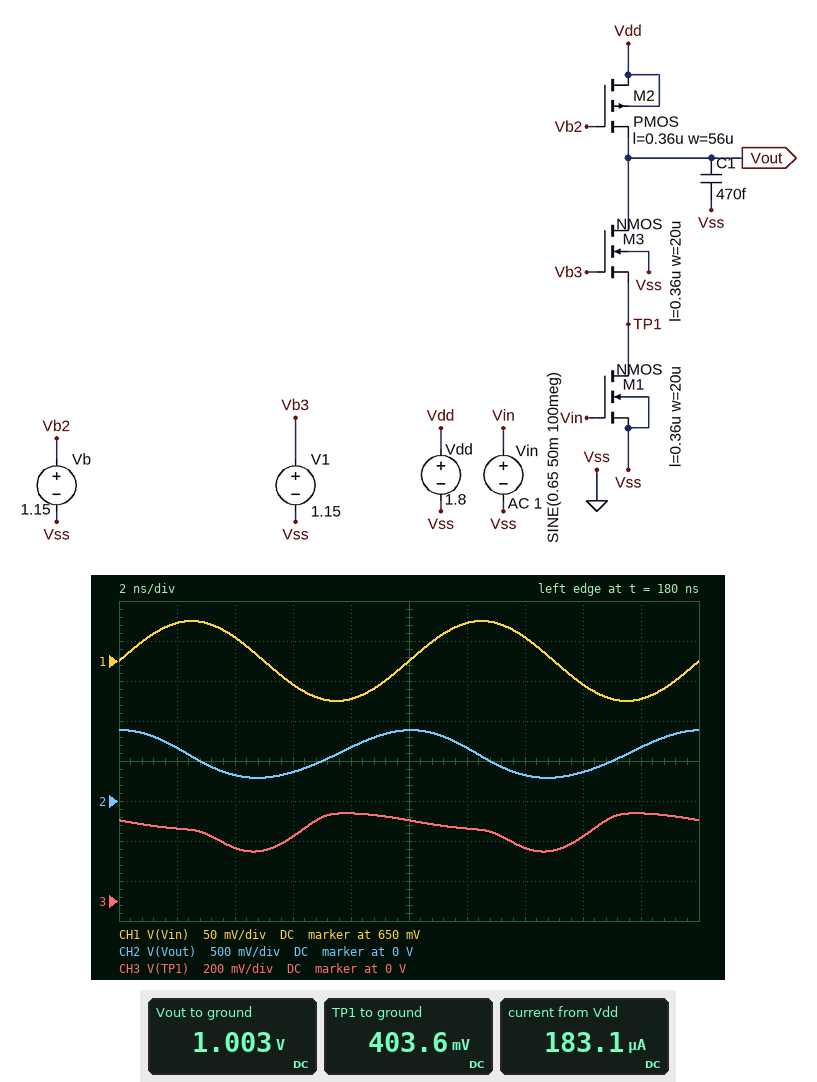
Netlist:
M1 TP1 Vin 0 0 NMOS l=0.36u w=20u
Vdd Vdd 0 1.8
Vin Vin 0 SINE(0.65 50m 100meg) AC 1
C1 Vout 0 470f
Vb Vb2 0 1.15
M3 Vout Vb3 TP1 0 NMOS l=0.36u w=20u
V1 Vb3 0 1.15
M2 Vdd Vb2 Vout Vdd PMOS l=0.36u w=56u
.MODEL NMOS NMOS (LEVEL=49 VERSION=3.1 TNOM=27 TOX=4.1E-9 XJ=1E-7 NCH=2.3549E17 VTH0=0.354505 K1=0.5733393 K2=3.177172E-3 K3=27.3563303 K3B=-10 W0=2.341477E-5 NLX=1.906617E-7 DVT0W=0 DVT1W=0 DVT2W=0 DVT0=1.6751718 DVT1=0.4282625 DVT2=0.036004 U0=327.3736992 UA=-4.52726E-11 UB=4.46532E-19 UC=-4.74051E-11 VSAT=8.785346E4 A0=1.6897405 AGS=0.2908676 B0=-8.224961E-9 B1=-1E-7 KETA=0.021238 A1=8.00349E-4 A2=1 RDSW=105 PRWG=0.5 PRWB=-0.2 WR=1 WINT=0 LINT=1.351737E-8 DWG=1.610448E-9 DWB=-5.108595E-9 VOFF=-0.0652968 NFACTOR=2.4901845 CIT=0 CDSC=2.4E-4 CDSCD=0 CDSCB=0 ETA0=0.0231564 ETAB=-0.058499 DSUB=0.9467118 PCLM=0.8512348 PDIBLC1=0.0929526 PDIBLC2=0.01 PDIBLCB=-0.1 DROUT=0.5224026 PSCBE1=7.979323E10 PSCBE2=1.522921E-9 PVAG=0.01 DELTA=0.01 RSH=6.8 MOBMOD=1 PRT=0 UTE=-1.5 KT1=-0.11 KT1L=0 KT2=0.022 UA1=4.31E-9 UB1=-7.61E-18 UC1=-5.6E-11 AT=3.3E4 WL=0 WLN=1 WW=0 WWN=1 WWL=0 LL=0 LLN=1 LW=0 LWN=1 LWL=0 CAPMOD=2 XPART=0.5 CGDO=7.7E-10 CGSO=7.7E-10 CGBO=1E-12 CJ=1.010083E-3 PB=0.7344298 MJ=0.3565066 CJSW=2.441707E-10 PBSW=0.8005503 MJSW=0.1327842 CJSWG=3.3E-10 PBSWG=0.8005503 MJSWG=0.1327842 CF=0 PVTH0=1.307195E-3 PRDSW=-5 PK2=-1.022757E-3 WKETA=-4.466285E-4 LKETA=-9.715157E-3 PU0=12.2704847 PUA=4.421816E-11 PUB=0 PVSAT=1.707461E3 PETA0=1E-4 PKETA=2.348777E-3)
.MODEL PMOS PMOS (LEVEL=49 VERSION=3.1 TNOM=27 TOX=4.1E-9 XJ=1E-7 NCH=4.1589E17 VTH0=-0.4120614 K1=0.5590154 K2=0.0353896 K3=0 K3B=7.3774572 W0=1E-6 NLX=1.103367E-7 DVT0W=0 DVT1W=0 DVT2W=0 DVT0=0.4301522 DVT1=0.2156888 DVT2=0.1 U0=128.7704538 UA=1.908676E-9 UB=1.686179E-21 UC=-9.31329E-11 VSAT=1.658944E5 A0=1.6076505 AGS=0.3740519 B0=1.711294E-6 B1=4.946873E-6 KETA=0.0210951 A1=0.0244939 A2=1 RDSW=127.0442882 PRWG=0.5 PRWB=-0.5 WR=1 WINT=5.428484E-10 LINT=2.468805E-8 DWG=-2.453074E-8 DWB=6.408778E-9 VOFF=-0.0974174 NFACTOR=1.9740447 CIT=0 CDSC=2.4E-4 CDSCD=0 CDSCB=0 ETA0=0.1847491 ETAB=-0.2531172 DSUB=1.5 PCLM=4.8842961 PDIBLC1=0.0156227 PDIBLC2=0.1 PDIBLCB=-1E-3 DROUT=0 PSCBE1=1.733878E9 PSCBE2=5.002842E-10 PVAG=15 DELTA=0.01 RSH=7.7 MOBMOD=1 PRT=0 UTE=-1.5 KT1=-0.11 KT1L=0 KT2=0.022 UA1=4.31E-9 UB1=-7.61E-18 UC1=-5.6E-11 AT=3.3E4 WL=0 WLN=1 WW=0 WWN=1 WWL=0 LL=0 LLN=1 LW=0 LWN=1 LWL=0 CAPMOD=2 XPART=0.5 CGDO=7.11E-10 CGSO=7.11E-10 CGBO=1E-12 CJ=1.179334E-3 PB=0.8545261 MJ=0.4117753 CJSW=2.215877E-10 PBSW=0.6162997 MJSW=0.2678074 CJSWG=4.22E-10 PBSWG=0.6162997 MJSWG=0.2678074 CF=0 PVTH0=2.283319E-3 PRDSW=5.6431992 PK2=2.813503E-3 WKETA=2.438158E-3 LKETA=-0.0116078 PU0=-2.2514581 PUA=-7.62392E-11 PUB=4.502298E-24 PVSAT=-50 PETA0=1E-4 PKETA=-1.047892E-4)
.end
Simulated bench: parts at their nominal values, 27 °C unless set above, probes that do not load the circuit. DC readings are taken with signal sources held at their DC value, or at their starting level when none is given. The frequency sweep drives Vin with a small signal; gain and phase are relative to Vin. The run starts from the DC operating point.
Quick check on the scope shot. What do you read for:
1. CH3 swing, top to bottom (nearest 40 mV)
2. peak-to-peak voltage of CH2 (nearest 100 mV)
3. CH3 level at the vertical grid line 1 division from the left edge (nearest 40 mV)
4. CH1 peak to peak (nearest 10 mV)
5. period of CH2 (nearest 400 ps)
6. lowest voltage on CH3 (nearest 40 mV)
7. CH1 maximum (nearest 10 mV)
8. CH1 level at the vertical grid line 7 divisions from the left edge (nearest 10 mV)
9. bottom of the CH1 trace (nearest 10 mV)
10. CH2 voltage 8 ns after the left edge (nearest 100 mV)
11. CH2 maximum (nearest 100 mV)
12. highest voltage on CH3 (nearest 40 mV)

200 mV
600 mV
360 mV
100 mV
10.0 ns
240 mV
700 mV
680 mV
600 mV
700 mV
900 mV
440 mV
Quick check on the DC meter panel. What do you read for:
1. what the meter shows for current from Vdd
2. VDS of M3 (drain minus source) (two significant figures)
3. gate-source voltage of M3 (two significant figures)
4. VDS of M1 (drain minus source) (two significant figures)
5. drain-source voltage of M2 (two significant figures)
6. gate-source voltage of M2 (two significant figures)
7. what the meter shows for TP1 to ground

183.1 µA
600 mV
750 mV
400 mV
800 mV
150 mV
403.6 mV
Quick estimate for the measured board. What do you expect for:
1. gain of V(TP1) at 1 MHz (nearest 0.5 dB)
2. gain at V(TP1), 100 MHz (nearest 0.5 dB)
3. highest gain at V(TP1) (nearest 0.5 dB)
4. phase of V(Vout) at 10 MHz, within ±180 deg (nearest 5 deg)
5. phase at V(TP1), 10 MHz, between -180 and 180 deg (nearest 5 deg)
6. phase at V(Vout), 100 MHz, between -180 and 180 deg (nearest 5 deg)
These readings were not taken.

5.5 dB
-2.0 dB
5.5 dB
115 deg
155 deg
90 deg
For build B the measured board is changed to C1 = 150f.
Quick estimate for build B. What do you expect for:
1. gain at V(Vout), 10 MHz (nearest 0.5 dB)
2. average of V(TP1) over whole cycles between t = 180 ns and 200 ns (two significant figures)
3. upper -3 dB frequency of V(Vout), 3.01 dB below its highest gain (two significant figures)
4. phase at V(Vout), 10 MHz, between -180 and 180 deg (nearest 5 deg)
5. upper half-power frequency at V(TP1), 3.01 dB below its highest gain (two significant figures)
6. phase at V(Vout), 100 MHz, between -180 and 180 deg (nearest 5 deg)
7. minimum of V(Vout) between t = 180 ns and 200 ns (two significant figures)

40.0 dB
340 mV
11 MHz
140 deg
14 MHz
95 deg
170 mV
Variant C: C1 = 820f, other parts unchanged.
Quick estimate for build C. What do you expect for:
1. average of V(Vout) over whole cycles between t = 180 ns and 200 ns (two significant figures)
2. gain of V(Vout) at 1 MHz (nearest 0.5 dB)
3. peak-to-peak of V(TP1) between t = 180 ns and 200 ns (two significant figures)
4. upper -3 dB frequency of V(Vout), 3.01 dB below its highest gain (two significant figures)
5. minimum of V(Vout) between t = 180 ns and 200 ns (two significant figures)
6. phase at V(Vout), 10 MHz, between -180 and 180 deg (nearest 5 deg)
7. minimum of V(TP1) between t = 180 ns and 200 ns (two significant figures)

540 mV
42.0 dB
130 mV
2.9 MHz
360 mV
105 deg
300 mV
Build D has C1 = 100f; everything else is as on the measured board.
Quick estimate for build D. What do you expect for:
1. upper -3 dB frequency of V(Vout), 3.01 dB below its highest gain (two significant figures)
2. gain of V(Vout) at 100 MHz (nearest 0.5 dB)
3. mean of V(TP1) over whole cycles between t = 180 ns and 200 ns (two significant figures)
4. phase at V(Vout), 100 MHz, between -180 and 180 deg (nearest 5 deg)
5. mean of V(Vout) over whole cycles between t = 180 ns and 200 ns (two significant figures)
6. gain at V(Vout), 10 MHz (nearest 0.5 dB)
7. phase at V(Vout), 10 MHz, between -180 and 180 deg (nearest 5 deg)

14 MHz
25.5 dB
330 mV
95 deg
850 mV
41.0 dB
145 deg
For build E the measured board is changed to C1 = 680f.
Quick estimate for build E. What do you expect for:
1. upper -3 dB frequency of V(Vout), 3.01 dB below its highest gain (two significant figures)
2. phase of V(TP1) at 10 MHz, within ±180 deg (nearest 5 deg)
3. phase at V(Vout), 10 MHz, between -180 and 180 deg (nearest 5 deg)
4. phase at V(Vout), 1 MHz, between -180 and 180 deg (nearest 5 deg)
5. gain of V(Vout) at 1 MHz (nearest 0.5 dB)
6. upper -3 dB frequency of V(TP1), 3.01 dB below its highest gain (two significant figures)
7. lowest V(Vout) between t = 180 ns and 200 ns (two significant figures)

3.4 MHz
160 deg
110 deg
165 deg
42.0 dB
4.2 MHz
340 mV
